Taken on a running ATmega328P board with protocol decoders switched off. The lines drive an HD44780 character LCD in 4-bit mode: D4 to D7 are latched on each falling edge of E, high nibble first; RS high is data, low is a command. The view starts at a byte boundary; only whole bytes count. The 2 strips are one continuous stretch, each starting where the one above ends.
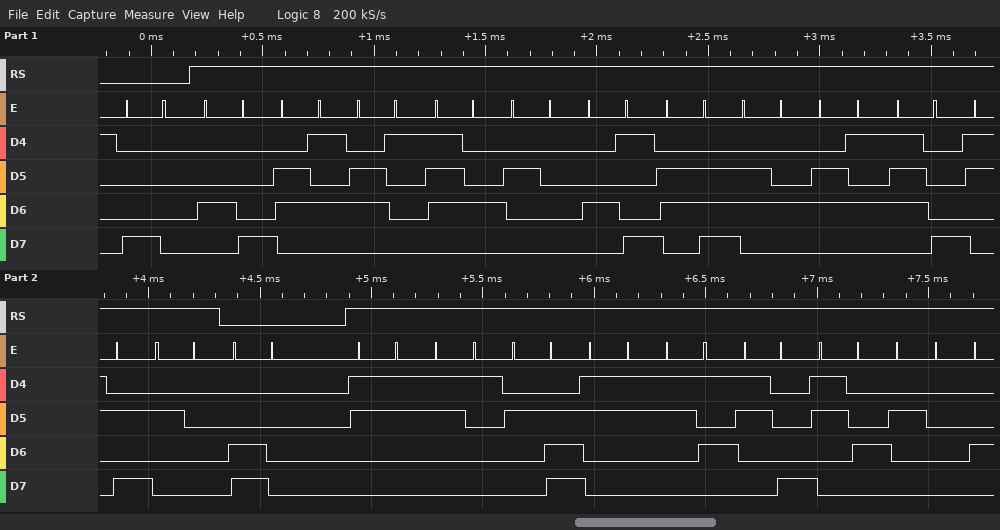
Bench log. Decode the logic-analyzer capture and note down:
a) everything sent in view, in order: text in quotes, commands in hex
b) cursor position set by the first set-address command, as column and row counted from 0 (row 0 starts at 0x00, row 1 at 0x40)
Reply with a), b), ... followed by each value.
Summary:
a) 0x80 "Heat Index: " 0xC0 "31.3584 "
b) column 0, row 0
